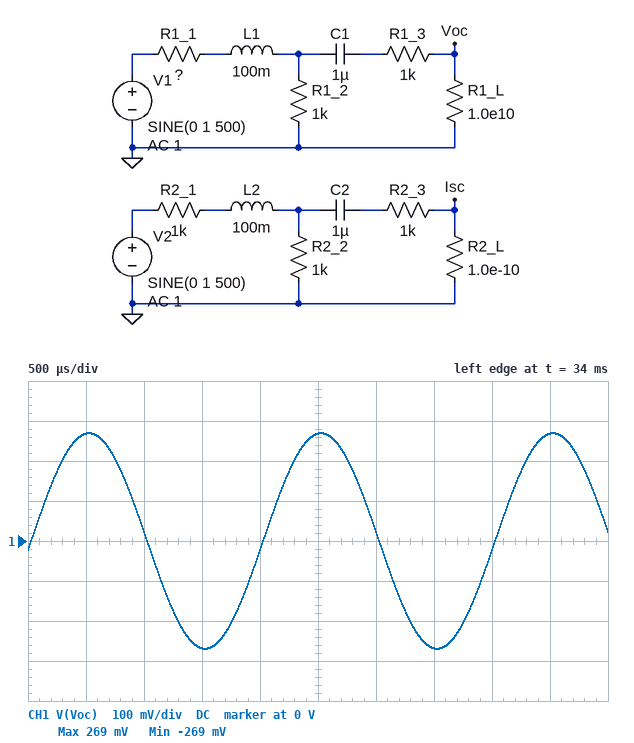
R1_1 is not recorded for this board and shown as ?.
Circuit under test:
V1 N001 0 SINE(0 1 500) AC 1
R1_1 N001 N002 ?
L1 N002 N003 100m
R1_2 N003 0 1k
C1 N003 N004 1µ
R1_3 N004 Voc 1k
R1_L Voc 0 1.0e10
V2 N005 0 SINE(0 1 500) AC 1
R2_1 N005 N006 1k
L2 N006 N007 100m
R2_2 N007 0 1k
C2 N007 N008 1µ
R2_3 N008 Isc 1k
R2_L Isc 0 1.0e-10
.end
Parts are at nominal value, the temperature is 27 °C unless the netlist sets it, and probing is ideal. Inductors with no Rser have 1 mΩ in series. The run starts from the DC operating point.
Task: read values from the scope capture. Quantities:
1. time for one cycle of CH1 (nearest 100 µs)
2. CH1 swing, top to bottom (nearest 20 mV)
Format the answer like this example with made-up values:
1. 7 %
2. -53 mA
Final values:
1. 2.0 ms
2. 540 mV
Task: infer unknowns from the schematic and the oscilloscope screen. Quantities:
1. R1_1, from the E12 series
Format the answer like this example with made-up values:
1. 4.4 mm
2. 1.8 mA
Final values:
1. 2.7 kΩ
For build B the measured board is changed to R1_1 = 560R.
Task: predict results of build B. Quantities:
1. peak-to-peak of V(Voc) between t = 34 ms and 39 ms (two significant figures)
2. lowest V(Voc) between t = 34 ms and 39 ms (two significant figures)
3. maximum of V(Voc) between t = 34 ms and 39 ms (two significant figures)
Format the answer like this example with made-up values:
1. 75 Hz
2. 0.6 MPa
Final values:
1. 1.3 V
2. -630 mV
3. 630 mV
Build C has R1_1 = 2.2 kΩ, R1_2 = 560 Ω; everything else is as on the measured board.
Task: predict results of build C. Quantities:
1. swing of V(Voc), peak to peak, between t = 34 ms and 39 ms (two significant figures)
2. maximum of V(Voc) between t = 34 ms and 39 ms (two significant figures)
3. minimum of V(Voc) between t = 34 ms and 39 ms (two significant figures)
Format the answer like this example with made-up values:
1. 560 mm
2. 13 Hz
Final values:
1. 400 mV
2. 200 mV
3. -200 mV
